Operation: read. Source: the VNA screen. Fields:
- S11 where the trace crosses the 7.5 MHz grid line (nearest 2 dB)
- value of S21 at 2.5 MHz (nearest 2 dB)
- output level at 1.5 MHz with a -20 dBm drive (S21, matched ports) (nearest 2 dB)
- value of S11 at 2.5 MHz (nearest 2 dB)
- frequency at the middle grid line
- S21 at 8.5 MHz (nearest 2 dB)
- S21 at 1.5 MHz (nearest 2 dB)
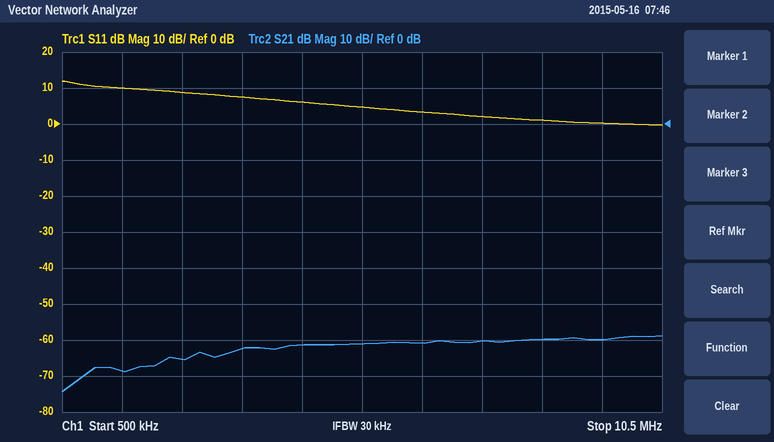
2 dB
-66 dB
-88 dBm
8 dB
5.5 MHz
-60 dB
-68 dB
